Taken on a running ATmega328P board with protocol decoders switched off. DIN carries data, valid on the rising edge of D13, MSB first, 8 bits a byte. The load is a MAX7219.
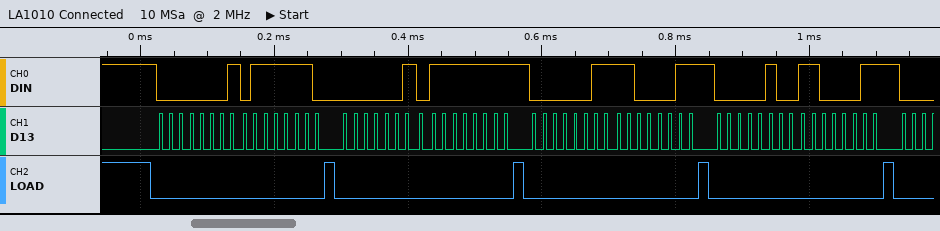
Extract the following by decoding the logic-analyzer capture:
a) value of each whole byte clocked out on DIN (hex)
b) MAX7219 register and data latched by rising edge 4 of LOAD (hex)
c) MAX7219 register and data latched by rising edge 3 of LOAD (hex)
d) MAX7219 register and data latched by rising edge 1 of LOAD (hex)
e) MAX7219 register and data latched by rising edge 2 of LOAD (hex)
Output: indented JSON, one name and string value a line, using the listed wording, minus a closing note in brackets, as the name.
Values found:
{
  "value of each whole byte clocked out on DIN": "01 7E 02 FF 03 C3 04 C3",
  "MAX7219 register and data latched by rising edge 4 of LOAD": "register 0x4, data 0xC3",
  "MAX7219 register and data latched by rising edge 3 of LOAD": "register 0x3, data 0xC3",
  "MAX7219 register and data latched by rising edge 1 of LOAD": "register 0x1, data 0x7E",
  "MAX7219 register and data latched by rising edge 2 of LOAD": "register 0x2, data 0xFF"
}
